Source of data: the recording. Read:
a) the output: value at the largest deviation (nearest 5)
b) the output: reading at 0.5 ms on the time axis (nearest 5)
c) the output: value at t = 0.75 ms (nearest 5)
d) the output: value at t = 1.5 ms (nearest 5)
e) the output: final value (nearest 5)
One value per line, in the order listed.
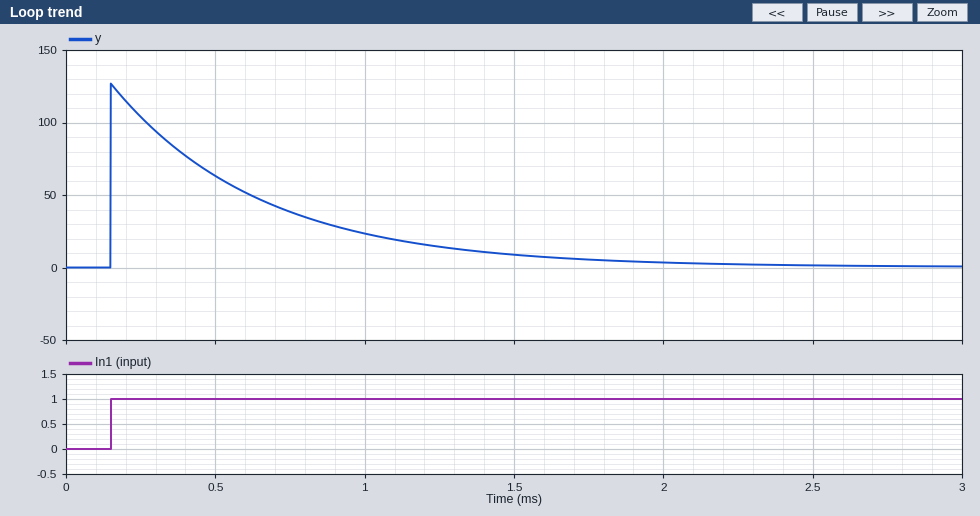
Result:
125
65
40
10
0
